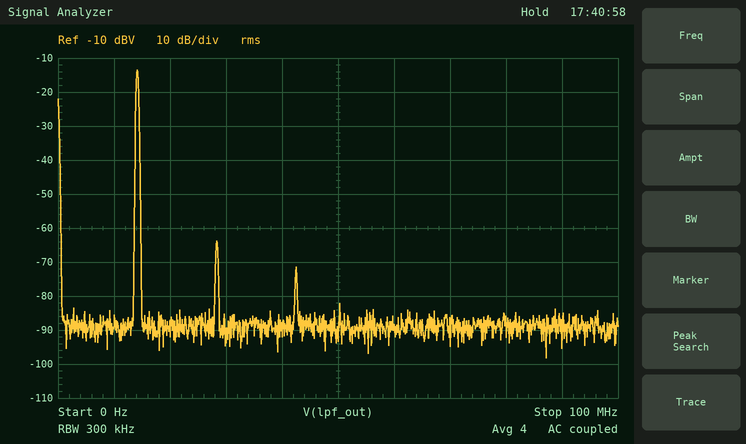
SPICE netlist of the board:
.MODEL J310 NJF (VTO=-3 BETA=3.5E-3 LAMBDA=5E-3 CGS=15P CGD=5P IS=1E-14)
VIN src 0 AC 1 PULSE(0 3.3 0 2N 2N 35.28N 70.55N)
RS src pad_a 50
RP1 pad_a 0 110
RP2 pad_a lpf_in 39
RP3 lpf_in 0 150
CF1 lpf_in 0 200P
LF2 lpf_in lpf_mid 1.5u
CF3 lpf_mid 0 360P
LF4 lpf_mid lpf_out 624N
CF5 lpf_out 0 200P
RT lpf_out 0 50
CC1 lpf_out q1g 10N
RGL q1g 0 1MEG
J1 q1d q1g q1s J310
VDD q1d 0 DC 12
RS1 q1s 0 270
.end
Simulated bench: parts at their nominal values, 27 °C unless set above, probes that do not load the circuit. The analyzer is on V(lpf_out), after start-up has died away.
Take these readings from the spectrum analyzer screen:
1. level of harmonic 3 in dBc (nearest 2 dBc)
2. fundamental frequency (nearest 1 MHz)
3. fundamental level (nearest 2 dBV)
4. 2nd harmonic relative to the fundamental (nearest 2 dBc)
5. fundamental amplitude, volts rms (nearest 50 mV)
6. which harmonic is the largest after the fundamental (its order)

-58 dBc
14 MHz
-14 dBV
-50 dBc
200 mV
2
